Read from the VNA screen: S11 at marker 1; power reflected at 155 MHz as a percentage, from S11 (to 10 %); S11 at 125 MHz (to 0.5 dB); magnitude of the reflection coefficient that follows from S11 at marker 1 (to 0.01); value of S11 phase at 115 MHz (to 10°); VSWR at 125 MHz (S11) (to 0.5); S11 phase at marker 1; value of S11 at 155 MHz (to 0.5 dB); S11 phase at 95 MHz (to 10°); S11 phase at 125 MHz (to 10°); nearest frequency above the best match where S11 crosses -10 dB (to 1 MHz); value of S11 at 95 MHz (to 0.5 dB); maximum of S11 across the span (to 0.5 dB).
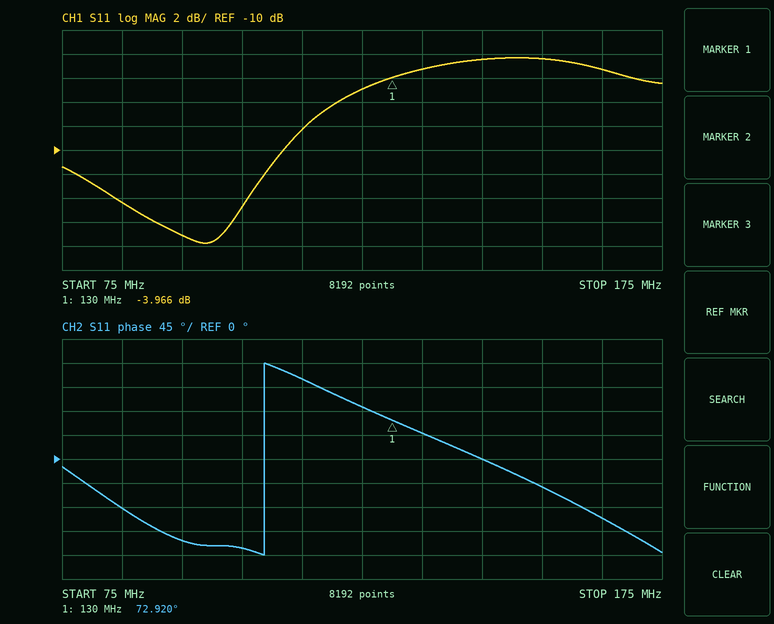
-3.966 dB
60 %
-5.0 dB
0.63
150°
3.5
72.920°
-2.5 dB
-150°
100°
112 MHz
-17.0 dB
-2.5 dB
